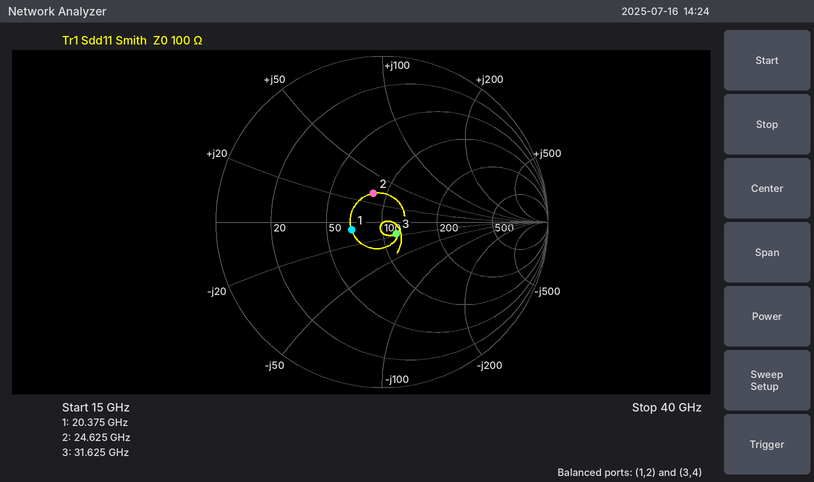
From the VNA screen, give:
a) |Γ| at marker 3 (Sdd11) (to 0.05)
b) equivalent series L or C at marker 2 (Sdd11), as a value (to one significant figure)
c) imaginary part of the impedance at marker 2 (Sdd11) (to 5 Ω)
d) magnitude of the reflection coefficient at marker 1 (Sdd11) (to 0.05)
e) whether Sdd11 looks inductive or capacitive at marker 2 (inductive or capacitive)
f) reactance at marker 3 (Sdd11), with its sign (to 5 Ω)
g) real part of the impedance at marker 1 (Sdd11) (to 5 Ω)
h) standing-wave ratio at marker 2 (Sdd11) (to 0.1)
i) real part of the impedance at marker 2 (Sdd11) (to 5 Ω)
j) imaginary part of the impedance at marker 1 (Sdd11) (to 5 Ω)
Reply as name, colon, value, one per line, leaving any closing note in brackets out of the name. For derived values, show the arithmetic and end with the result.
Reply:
|Γ| at marker 3 (Sdd11): 0.10
equivalent series L or C at marker 2 (Sdd11), as a value: L = 30 Ω/(2π × 24.625 GHz) ≈ 194 pH, so 200 pH to one significant figure
imaginary part of the impedance at marker 2 (Sdd11): +30 Ω
magnitude of the reflection coefficient at marker 1 (Sdd11): 0.20
whether Sdd11 looks inductive or capacitive at marker 2: inductive
reactance at marker 3 (Sdd11), with its sign: -15 Ω
real part of the impedance at marker 1 (Sdd11): 70 Ω
standing-wave ratio at marker 2 (Sdd11): 1.4
real part of the impedance at marker 2 (Sdd11): 85 Ω
imaginary part of the impedance at marker 1 (Sdd11): -5 Ω
